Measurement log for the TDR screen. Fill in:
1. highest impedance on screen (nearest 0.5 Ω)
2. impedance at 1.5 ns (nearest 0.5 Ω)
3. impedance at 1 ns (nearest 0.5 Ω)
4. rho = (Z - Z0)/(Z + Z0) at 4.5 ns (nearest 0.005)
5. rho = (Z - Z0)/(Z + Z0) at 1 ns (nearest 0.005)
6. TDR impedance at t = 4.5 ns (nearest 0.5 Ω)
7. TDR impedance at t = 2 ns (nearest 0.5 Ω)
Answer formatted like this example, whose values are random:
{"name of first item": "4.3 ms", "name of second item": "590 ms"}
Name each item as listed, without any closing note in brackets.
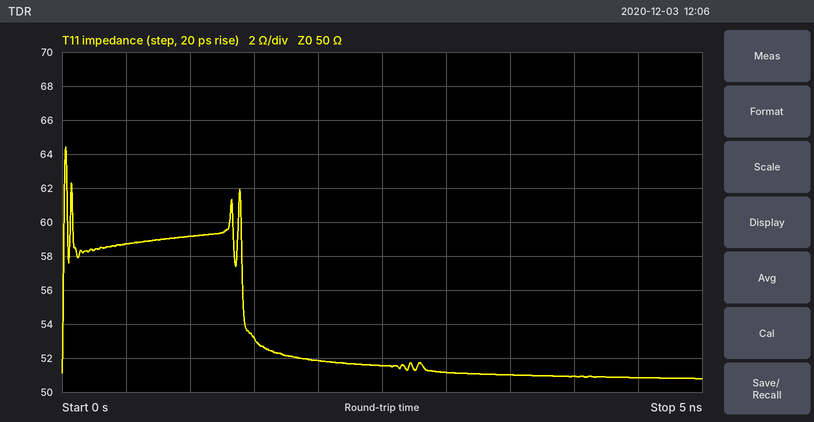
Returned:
{"highest impedance on screen": "64.5 Ω", "impedance at 1.5 ns": "53.0 Ω", "impedance at 1 ns": "59.0 Ω", "rho = (Z - Z0)/(Z + Z0) at 4.5 ns": "+0.010", "rho = (Z - Z0)/(Z + Z0) at 1 ns": "+0.085", "TDR impedance at t = 4.5 ns": "51.0 Ω", "TDR impedance at t = 2 ns": "52.0 Ω"}
